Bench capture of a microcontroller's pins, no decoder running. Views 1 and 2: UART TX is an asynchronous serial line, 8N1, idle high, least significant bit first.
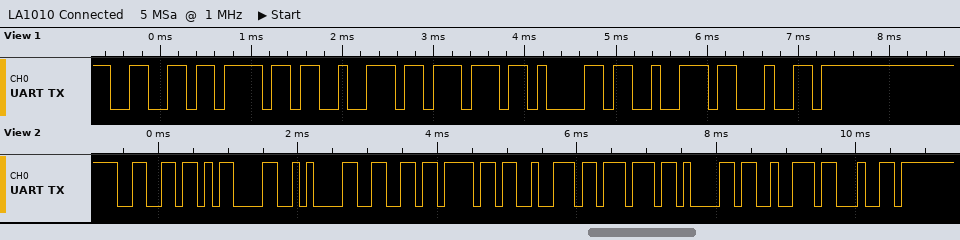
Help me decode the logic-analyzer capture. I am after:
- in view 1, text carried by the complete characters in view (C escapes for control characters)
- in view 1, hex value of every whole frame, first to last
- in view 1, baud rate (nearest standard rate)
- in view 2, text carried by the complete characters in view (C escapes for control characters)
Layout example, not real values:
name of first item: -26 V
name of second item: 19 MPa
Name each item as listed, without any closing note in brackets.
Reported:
in view 1, text carried by the complete characters in view: "forward"
in view 1, hex value of every whole frame, first to last: 66 6F 72 77 61 72 64
in view 1, baud rate: 9600 baud
in view 2, text carried by the complete characters in view: "f\r\nforward"
